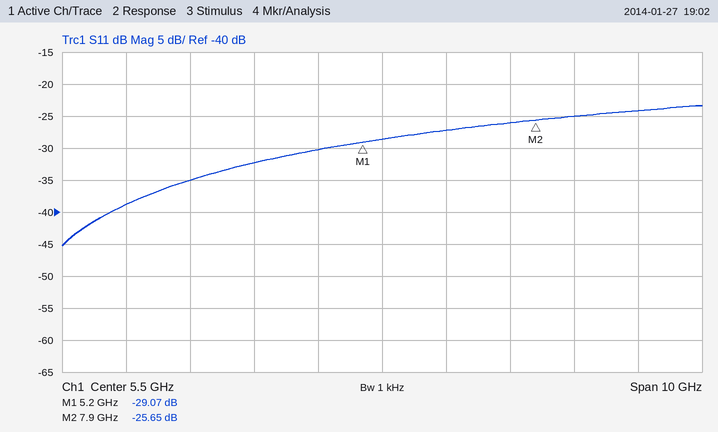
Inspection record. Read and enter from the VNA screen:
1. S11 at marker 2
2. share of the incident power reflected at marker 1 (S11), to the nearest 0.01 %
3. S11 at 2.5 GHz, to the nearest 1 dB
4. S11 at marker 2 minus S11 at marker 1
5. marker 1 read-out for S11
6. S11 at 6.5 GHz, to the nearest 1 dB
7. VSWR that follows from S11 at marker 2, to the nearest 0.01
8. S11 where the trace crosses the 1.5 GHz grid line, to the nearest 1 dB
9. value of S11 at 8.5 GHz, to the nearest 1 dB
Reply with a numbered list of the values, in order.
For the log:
1. -25.65 dB
2. 0.12 %
3. -35 dB
4. 3.42 dB
5. -29.07 dB
6. -27 dB
7. 1.11
8. -39 dB
9. -25 dB
